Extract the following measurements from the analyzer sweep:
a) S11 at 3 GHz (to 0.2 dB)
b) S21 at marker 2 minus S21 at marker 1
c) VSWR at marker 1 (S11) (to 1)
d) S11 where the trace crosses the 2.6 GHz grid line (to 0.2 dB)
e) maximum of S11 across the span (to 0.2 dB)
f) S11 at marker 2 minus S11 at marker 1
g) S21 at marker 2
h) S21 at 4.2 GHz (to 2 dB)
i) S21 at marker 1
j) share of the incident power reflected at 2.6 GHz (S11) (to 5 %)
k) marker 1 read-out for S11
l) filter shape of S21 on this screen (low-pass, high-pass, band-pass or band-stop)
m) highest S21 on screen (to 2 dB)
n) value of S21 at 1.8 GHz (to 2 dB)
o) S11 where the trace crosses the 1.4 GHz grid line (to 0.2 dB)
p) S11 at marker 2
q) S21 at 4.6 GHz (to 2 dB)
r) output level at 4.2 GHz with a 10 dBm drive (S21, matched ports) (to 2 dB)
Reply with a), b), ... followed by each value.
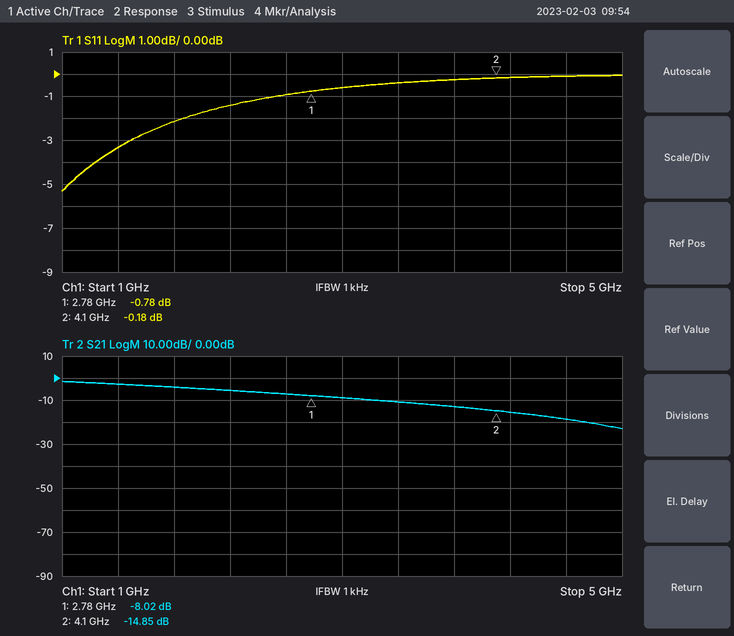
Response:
a) -0.6 dB
b) -6.83 dB
c) 22
d) -1.0 dB
e) 0.0 dB
f) 0.60 dB
g) -14.85 dB
h) -16 dB
i) -8.02 dB
j) 80 %
k) -0.78 dB
l) low-pass
m) -2 dB
n) -4 dB
o) -3.4 dB
p) -0.18 dB
q) -18 dB
r) -6 dBm
